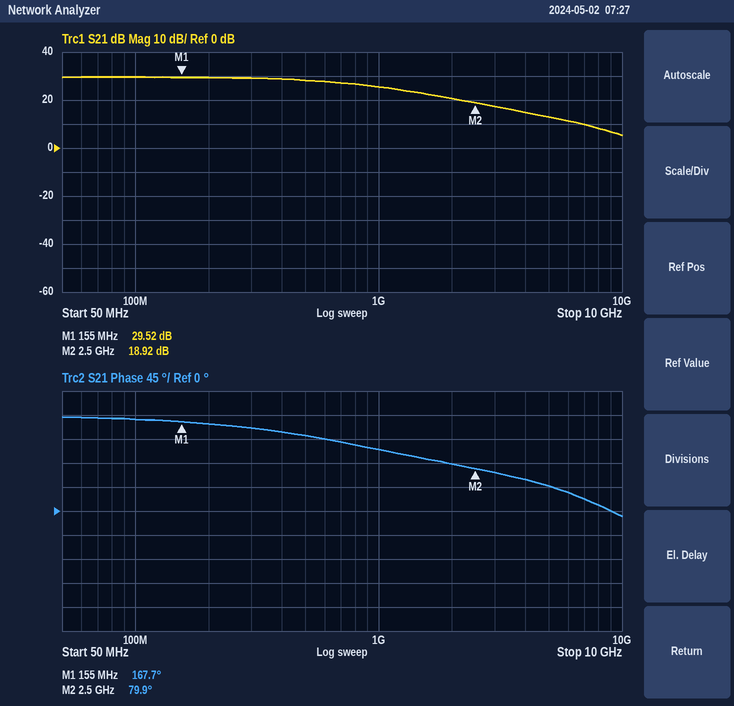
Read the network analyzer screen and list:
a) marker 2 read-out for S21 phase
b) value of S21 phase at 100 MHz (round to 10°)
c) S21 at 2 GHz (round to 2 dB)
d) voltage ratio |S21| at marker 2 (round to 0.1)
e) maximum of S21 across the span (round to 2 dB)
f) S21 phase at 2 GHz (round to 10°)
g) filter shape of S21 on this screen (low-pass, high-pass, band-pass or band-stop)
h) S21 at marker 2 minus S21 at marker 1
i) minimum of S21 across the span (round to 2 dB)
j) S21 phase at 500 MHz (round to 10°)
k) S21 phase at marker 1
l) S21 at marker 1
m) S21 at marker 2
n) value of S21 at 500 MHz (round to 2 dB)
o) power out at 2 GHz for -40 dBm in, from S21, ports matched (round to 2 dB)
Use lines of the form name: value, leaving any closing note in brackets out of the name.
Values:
marker 2 read-out for S21 phase: 79.9°
value of S21 phase at 100 MHz: 170°
S21 at 2 GHz: 20 dB
voltage ratio |S21| at marker 2: 8.8
maximum of S21 across the span: 30 dB
S21 phase at 2 GHz: 90°
filter shape of S21 on this screen: low-pass
S21 at marker 2 minus S21 at marker 1: -10.60 dB
minimum of S21 across the span: 6 dB
S21 phase at 500 MHz: 140°
S21 phase at marker 1: 167.7°
S21 at marker 1: 29.52 dB
S21 at marker 2: 18.92 dB
value of S21 at 500 MHz: 28 dB
power out at 2 GHz for -40 dBm in, from S21, ports matched: -20 dBm
